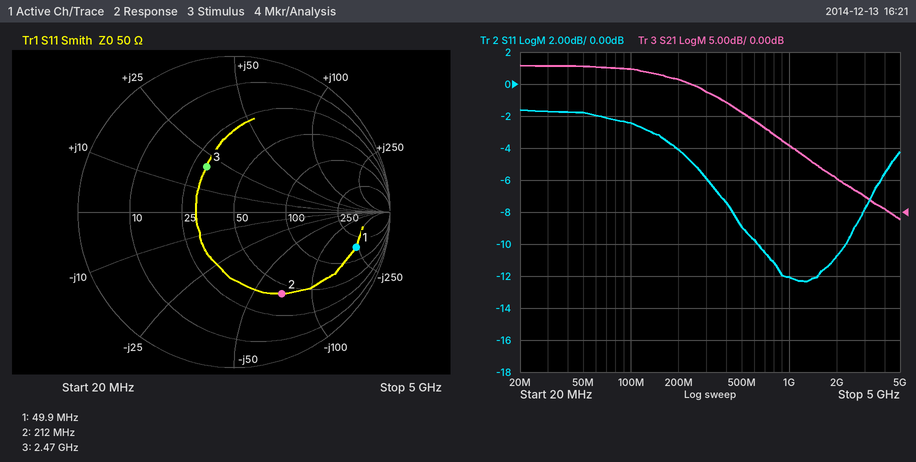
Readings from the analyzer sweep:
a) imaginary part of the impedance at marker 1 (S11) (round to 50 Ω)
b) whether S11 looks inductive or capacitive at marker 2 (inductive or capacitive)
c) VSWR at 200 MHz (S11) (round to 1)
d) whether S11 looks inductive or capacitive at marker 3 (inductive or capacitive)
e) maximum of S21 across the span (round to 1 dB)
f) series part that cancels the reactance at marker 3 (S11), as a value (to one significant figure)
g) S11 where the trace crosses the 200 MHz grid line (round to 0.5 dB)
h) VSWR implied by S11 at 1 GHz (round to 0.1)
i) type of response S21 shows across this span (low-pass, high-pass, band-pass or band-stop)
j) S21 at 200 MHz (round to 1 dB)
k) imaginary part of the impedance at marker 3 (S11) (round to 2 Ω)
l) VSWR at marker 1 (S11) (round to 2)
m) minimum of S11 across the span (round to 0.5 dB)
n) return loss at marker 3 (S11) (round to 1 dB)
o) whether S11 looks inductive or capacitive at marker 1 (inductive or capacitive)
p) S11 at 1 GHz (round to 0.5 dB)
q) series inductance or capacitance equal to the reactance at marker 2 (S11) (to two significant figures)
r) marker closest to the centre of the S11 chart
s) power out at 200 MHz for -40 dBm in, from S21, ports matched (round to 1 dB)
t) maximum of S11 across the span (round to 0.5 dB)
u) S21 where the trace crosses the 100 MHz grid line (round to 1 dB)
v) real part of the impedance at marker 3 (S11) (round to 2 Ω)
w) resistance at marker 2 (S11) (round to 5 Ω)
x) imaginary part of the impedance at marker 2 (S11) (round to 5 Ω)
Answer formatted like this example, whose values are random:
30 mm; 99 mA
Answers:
-250 Ω; capacitive; 4; inductive; 23 dB; 3 pF; -4.0 dB; 1.7; low-pass; 21 dB; +20 Ω; 10; -12.5 dB; 9 dB; capacitive; -12.0 dB; 11 pF; marker 3; -19 dBm; -1.5 dB; 22 dB; 30 Ω; 40 Ω; -70 Ω
